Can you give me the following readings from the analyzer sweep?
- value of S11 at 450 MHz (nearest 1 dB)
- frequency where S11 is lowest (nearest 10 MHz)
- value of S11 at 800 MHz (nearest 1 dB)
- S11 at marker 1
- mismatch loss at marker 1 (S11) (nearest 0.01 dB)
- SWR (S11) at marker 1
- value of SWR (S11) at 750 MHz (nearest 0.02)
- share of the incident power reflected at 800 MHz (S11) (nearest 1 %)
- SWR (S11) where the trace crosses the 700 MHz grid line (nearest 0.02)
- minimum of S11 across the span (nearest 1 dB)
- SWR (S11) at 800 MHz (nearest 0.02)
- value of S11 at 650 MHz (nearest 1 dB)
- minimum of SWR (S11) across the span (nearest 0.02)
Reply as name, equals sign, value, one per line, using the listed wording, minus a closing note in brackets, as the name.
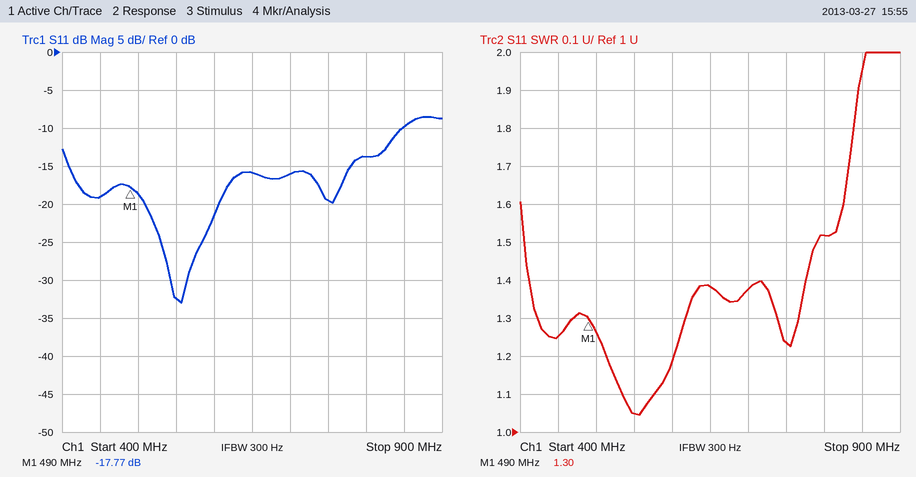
value of S11 at 450 MHz = -19 dB
frequency where S11 is lowest = 560 MHz
value of S11 at 800 MHz = -14 dB
S11 at marker 1 = -17.77 dB
mismatch loss at marker 1 (S11) = 0.07 dB
SWR (S11) at marker 1 = 1.30
value of SWR (S11) at 750 MHz = 1.24
share of the incident power reflected at 800 MHz (S11) = 4 %
SWR (S11) where the trace crosses the 700 MHz grid line = 1.38
minimum of S11 across the span = -33 dB
SWR (S11) at 800 MHz = 1.52
value of S11 at 650 MHz = -16 dB
minimum of SWR (S11) across the span = 1.04
